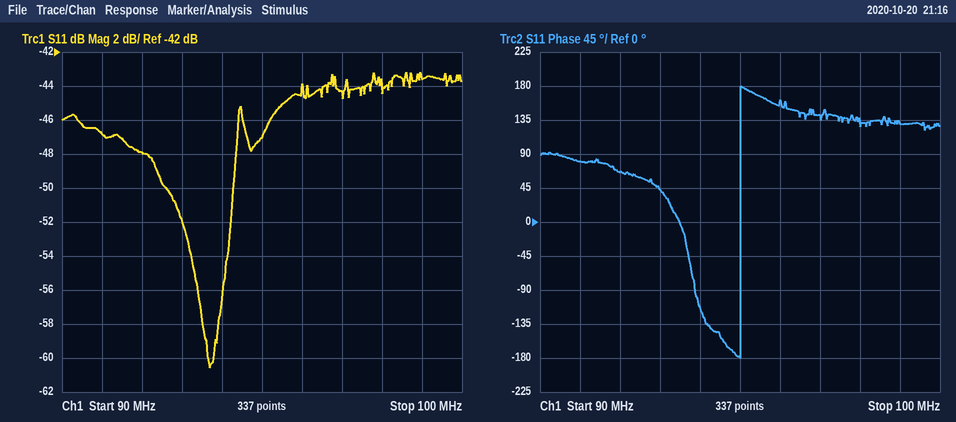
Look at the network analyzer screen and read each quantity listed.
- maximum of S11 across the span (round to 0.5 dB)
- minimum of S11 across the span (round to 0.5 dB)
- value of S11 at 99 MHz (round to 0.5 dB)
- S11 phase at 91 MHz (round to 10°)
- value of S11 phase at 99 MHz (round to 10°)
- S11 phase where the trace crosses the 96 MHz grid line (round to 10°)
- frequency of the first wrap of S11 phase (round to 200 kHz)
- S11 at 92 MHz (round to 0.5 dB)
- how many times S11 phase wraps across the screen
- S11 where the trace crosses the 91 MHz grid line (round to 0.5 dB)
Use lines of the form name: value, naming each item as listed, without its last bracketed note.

maximum of S11 across the span: -43.0 dB
minimum of S11 across the span: -60.5 dB
value of S11 at 99 MHz: -43.5 dB
S11 phase at 91 MHz: 80°
value of S11 phase at 99 MHz: 130°
S11 phase where the trace crosses the 96 MHz grid line: 160°
frequency of the first wrap of S11 phase: 95.0 MHz
S11 at 92 MHz: -48.0 dB
how many times S11 phase wraps across the screen: 1
S11 where the trace crosses the 91 MHz grid line: -47.0 dB
